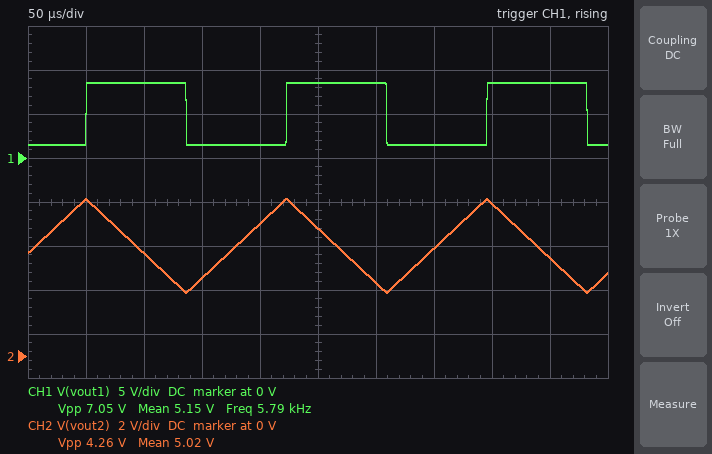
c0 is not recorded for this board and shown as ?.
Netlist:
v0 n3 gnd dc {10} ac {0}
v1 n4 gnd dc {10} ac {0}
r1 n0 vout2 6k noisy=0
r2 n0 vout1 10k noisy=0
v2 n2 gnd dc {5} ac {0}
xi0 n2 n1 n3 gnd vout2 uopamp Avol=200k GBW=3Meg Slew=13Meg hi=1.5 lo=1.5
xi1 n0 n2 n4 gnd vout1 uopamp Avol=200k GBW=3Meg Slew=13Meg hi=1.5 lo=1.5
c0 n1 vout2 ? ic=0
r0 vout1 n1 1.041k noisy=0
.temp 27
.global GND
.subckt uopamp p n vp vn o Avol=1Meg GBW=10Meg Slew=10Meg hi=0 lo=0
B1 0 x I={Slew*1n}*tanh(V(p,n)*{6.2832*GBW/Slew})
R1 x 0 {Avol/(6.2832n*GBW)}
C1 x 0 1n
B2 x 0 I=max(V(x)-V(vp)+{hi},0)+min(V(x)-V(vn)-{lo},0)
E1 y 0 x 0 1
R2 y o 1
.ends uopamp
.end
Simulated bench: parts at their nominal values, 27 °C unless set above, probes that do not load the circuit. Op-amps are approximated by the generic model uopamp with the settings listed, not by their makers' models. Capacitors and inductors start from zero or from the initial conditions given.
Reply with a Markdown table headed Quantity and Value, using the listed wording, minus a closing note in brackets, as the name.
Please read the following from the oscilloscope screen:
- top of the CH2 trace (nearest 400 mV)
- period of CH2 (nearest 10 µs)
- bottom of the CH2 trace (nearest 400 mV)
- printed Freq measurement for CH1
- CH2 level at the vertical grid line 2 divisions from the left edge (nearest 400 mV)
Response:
| Quantity | Value |
|---|---|
| top of the CH2 trace | 7.2 V |
| period of CH2 | 170 µs |
| bottom of the CH2 trace | 2.8 V |
| printed Freq measurement for CH1 | 5.79 kHz |
| CH2 level at the vertical grid line 2 divisions from the left edge | 4.8 V |
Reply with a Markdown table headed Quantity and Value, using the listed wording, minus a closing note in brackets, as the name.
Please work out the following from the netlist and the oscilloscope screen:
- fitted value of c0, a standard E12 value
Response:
| Quantity | Value |
|---|---|
| fitted value of c0, a standard E12 value | 68 nF |
